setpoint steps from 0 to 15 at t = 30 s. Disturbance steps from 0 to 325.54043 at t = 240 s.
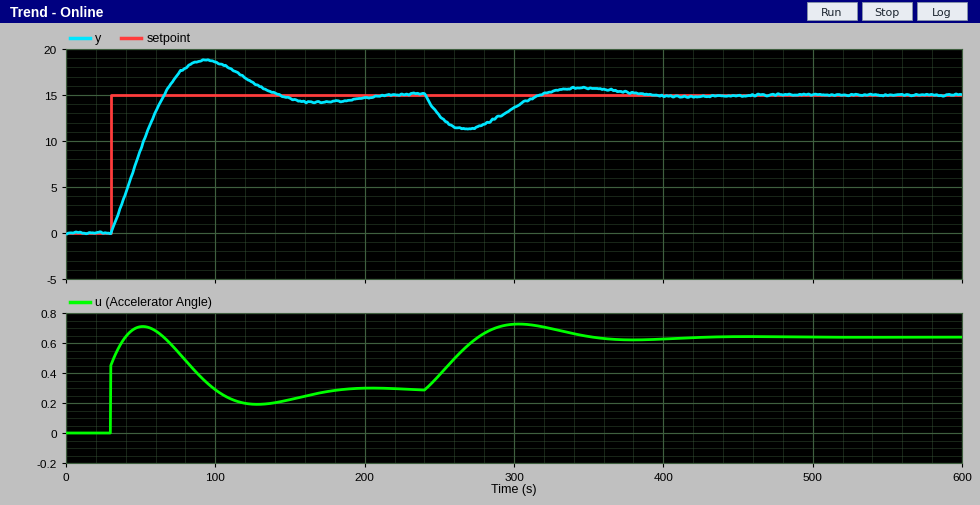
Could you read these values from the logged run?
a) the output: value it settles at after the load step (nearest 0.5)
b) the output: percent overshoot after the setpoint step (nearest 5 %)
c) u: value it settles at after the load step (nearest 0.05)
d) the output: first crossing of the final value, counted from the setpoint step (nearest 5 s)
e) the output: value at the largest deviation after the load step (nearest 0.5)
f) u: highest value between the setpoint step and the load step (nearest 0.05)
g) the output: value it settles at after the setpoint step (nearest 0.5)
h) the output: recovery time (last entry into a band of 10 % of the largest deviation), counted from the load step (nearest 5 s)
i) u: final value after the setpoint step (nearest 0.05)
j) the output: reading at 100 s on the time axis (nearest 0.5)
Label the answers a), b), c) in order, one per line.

a) 15.0
b) 25 %
c) 0.65
d) 35 s
e) 11.5
f) 0.70
g) 15.0
h) 130 s
i) 0.30
j) 18.5
